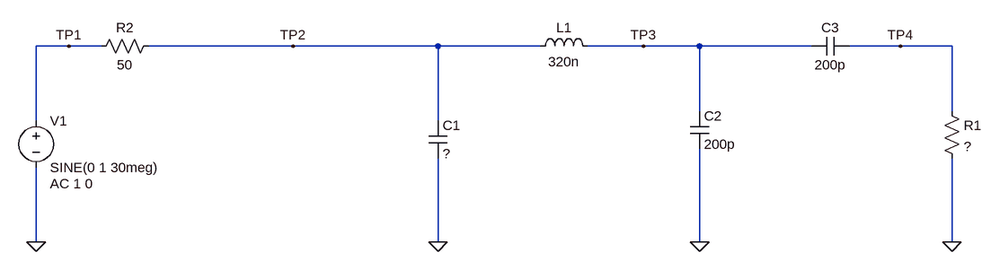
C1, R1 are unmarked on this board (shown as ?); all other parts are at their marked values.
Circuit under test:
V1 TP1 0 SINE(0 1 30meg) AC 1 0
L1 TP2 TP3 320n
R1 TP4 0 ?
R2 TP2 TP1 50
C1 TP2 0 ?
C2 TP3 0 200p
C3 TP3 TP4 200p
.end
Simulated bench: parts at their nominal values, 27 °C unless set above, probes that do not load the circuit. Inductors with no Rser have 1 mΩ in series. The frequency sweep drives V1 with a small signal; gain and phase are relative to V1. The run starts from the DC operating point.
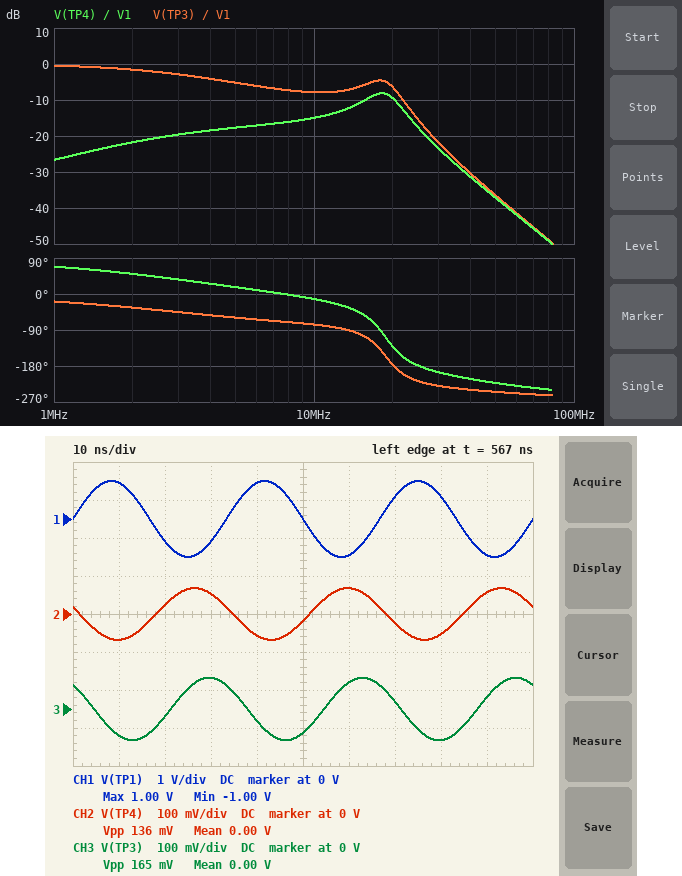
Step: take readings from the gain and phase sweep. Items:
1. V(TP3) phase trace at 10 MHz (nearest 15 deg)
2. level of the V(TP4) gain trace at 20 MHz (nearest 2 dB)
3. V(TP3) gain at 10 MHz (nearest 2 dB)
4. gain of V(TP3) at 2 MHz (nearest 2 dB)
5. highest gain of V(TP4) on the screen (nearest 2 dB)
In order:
-75 deg
-10 dB
-8 dB
-2 dB
-8 dB
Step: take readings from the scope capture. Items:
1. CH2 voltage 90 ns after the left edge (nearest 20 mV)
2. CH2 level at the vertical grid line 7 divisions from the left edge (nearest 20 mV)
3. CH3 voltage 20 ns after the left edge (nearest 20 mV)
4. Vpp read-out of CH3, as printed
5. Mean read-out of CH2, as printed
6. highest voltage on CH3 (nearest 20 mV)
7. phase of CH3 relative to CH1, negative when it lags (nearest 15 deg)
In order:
60 mV
-20 mV
-20 mV
165 mV
0.00 V
80 mV
135 deg
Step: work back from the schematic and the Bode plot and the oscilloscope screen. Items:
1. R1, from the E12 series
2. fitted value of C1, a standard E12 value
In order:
39 Ω
680 pF
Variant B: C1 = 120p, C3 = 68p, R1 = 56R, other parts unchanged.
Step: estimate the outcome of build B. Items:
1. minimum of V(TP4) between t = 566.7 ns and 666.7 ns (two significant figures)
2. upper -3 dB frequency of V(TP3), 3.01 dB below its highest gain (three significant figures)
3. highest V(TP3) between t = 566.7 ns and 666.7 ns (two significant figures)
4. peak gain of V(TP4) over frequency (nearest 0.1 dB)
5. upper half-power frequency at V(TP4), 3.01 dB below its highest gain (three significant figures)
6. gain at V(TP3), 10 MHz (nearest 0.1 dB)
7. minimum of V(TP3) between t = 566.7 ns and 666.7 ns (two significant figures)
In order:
-290 mV
12.9 MHz
500 mV
-9.9 dB
33.9 MHz
-2.3 dB
-500 mV
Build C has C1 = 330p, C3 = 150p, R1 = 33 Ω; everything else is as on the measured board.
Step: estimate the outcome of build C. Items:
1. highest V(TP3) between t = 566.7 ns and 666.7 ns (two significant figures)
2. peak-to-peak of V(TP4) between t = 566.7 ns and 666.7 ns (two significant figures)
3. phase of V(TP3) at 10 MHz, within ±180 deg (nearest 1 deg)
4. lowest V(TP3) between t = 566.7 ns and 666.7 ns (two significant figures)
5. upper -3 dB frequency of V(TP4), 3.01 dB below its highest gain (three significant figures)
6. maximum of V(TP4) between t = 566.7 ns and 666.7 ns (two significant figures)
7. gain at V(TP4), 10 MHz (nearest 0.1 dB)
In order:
190 mV
260 mV
-69 deg
-190 mV
24.7 MHz
130 mV
-15.8 dB
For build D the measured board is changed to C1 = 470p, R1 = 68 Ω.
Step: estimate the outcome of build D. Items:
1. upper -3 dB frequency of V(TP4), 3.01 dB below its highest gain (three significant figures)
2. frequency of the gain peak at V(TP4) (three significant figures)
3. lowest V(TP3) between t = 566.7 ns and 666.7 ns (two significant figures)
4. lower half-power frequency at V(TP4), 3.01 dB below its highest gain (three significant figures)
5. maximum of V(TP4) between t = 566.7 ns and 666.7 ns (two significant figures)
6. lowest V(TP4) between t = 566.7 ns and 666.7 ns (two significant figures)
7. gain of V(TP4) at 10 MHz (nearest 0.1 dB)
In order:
24.3 MHz
20.8 MHz
-170 mV
15.2 MHz
160 mV
-160 mV
-10.3 dB
